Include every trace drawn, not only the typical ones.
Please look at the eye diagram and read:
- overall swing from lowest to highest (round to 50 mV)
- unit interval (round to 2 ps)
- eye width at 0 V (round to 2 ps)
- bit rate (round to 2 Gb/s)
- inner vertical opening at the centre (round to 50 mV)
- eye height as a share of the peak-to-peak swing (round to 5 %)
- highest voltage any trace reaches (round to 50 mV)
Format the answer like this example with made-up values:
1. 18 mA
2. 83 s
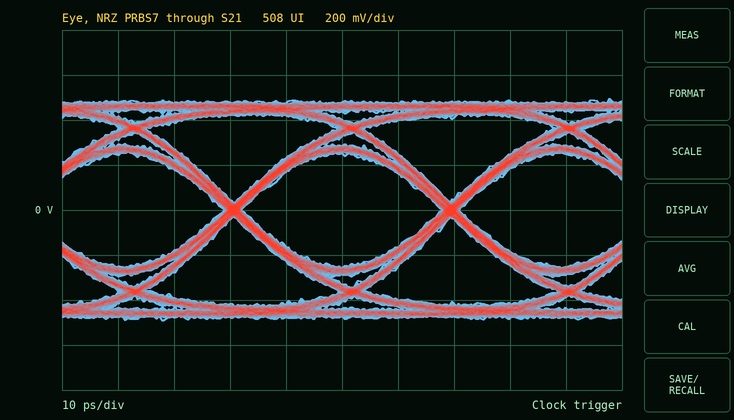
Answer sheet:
1. 1.00 V
2. 38 ps
3. 36 ps
4. 26 Gb/s
5. 500 mV
6. 50 %
7. 500 mV
